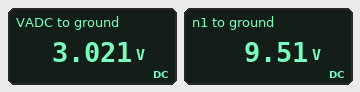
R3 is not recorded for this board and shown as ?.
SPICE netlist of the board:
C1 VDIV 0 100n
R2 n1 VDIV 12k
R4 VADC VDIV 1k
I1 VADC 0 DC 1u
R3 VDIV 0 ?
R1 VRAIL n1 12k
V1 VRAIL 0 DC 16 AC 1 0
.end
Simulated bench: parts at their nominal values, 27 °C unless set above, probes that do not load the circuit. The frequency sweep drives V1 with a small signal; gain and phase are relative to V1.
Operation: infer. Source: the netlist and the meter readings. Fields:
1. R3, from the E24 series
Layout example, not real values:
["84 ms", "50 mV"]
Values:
["5.6 kΩ"]
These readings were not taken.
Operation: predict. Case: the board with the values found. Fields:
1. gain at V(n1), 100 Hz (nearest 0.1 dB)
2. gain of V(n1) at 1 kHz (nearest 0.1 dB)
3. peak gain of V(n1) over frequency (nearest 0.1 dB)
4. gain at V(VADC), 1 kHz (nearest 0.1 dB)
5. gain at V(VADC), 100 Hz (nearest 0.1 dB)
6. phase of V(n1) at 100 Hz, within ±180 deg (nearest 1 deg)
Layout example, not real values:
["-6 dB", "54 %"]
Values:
["-4.6 dB", "-5.8 dB", "-4.5 dB", "-24.1 dB", "-14.8 dB", "-2 deg"]
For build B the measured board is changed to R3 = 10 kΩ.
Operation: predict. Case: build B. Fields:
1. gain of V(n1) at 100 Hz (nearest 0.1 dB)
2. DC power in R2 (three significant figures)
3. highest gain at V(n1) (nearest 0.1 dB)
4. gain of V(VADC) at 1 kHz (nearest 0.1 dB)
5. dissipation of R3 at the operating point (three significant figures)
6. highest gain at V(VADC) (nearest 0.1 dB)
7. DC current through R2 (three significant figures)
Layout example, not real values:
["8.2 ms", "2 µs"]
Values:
["-4.1 dB", "2.66 mW", "-3.8 dB", "-23.8 dB", "2.21 mW", "-10.6 dB", "471 µA"]
